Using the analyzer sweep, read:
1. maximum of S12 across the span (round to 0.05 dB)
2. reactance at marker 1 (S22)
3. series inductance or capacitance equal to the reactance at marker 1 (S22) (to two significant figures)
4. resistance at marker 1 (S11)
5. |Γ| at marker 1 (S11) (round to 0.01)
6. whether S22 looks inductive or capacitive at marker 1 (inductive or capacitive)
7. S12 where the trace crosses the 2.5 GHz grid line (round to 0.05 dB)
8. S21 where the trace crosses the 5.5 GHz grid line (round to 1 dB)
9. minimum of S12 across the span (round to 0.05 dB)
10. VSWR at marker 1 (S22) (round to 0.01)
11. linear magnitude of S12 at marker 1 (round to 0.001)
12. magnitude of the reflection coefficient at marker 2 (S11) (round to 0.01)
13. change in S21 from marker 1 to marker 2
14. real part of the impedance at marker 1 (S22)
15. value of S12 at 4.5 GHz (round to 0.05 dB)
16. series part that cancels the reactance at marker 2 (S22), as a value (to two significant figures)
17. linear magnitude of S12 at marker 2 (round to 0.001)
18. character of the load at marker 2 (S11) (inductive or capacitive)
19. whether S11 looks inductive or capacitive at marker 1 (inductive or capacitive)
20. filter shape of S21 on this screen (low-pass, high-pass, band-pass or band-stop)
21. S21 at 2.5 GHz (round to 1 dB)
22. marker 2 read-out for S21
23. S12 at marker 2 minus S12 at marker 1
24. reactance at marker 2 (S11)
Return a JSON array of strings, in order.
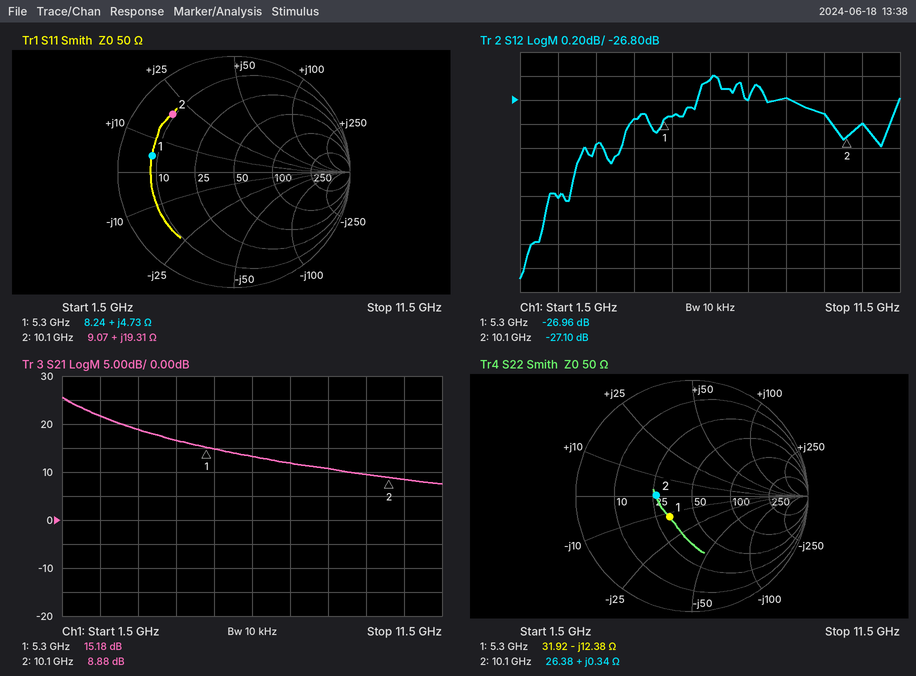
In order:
["-26.60 dB", "-12.38 Ω", "2.4 pF", "8.24 Ω", "0.72", "capacitive", "-27.60 dB", "15 dB", "-28.30 dB", "1.72", "0.045", "0.73", "-6.30 dB", "31.92 Ω", "-26.95 dB", "46 pF", "0.044", "inductive", "inductive", "low-pass", "22 dB", "8.88 dB", "-0.14 dB", "+19.31 Ω"]
